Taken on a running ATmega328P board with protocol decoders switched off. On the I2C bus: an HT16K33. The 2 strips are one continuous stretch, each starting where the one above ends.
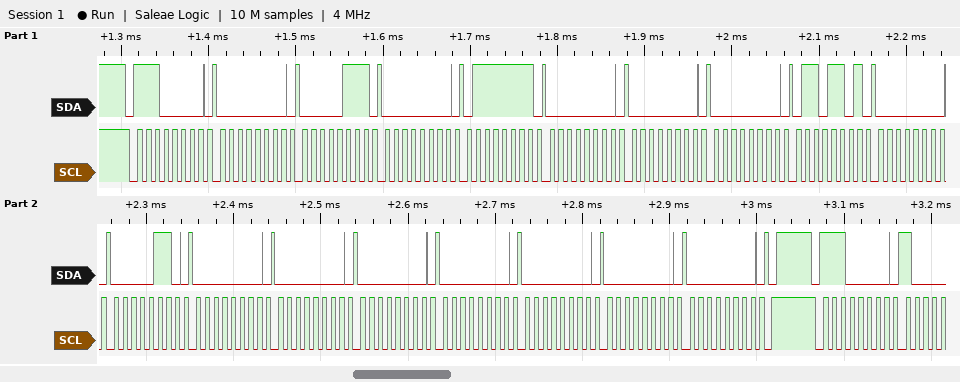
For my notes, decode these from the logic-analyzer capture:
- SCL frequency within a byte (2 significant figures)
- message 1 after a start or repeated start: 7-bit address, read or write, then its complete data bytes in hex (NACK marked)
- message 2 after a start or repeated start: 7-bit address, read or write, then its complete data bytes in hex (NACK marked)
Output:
100 kHz
0x70 write: 00 07 00 7F 00 00 00 6D 00 06 00 00 00 00 00 00 00
0x70 write
